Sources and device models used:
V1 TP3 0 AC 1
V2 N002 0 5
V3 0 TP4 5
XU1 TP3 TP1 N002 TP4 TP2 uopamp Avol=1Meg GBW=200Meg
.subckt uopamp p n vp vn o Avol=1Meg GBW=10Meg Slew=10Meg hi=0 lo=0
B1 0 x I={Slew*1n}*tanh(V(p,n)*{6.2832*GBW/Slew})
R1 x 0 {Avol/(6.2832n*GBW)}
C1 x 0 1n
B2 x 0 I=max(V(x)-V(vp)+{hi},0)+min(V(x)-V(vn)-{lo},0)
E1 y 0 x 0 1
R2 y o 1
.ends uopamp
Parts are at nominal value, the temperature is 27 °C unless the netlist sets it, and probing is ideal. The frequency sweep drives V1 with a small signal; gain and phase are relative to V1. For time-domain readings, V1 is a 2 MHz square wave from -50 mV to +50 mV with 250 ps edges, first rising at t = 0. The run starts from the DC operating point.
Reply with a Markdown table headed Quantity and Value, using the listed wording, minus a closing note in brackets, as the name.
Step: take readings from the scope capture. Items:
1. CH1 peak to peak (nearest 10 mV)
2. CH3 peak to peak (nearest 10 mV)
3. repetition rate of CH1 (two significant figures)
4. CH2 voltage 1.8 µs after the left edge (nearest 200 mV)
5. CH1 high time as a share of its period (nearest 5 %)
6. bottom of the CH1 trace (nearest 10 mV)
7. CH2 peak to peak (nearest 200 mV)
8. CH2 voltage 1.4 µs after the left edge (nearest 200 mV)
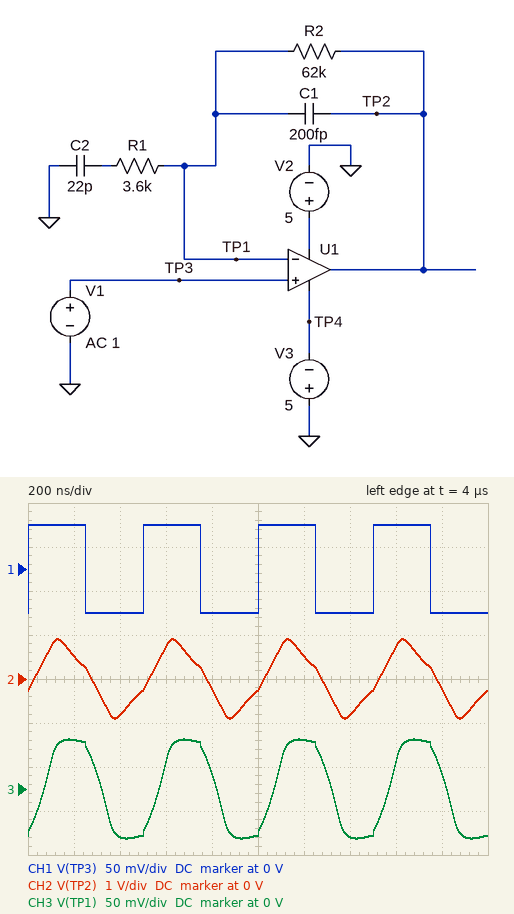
| Quantity | Value |
|---|---|
| CH1 peak to peak | 100 mV |
| CH3 peak to peak | 110 mV |
| repetition rate of CH1 | 2.0 MHz |
| CH2 voltage 1.8 µs after the left edge | -200 mV |
| CH1 high time as a share of its period | 50 % |
| bottom of the CH1 trace | -50 mV |
| CH2 peak to peak | 1.8 V |
| CH2 voltage 1.4 µs after the left edge | -800 mV |
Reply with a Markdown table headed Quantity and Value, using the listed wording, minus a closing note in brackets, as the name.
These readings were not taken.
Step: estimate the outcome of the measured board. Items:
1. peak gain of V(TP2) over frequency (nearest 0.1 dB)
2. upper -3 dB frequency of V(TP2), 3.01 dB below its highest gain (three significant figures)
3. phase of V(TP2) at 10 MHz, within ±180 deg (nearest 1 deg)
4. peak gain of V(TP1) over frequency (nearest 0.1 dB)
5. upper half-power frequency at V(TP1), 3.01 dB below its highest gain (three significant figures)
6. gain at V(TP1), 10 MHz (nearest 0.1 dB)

| Quantity | Value |
|---|---|
| peak gain of V(TP2) over frequency | 24.0 dB |
| upper -3 dB frequency of V(TP2), 3.01 dB below its highest gain | 8.39 MHz |
| phase of V(TP2) at 10 MHz, within ±180 deg | -51 deg |
| peak gain of V(TP1) over frequency | 0.6 dB |
| upper half-power frequency at V(TP1), 3.01 dB below its highest gain | 8.16 MHz |
| gain at V(TP1), 10 MHz | -3.2 dB |
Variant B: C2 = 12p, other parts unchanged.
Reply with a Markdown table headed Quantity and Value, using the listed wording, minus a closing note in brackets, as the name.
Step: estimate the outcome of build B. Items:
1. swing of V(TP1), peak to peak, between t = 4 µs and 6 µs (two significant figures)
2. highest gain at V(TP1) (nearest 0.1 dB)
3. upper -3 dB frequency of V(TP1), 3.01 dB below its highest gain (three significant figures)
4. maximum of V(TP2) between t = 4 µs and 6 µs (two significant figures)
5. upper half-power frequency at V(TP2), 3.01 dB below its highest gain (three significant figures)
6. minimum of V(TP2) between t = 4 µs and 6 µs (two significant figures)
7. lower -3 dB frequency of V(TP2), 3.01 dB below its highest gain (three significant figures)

| Quantity | Value |
|---|---|
| swing of V(TP1), peak to peak, between t = 4 µs and 6 µs | 120 mV |
| highest gain at V(TP1) | 0.8 dB |
| upper -3 dB frequency of V(TP1), 3.01 dB below its highest gain | 9.05 MHz |
| maximum of V(TP2) between t = 4 µs and 6 µs | 770 mV |
| upper half-power frequency at V(TP2), 3.01 dB below its highest gain | 9.95 MHz |
| minimum of V(TP2) between t = 4 µs and 6 µs | -770 mV |
| lower -3 dB frequency of V(TP2), 3.01 dB below its highest gain | 2.20 MHz |
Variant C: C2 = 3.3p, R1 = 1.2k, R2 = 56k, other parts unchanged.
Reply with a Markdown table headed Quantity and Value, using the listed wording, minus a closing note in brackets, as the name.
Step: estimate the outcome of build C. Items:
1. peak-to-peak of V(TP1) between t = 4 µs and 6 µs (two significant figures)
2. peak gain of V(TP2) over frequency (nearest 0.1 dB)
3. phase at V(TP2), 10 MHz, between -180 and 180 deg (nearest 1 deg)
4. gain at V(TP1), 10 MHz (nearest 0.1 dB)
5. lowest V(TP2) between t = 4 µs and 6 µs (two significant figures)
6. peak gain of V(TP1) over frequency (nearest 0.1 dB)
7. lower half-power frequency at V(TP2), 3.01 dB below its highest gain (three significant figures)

| Quantity | Value |
|---|---|
| peak-to-peak of V(TP1) between t = 4 µs and 6 µs | 140 mV |
| peak gain of V(TP2) over frequency | 22.1 dB |
| phase at V(TP2), 10 MHz, between -180 and 180 deg | 7 deg |
| gain at V(TP1), 10 MHz | 1.9 dB |
| lowest V(TP2) between t = 4 µs and 6 µs | -460 mV |
| peak gain of V(TP1) over frequency | 2.0 dB |
| lower half-power frequency at V(TP2), 3.01 dB below its highest gain | 6.57 MHz |
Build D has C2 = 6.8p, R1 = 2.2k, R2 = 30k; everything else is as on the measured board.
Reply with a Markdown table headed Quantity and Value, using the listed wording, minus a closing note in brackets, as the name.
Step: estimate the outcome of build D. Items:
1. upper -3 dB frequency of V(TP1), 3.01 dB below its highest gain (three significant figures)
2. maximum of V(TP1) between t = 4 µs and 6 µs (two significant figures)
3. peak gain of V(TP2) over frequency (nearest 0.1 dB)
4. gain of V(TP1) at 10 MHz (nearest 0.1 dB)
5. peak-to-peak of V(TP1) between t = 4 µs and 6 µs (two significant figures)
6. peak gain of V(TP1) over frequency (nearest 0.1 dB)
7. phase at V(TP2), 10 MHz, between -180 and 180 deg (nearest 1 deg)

| Quantity | Value |
|---|---|
| upper -3 dB frequency of V(TP1), 3.01 dB below its highest gain | 14.9 MHz |
| maximum of V(TP1) between t = 4 µs and 6 µs | 64 mV |
| peak gain of V(TP2) over frequency | 20.4 dB |
| gain of V(TP1) at 10 MHz | 0.7 dB |
| peak-to-peak of V(TP1) between t = 4 µs and 6 µs | 130 mV |
| peak gain of V(TP1) over frequency | 1.3 dB |
| phase at V(TP2), 10 MHz, between -180 and 180 deg | -5 deg |
